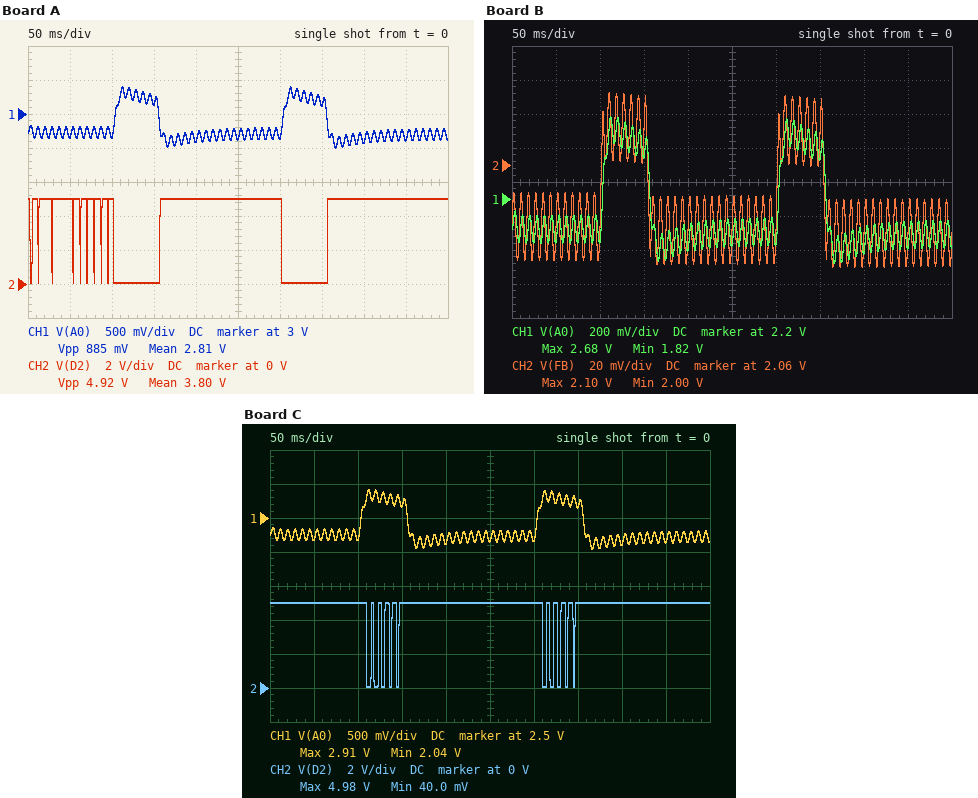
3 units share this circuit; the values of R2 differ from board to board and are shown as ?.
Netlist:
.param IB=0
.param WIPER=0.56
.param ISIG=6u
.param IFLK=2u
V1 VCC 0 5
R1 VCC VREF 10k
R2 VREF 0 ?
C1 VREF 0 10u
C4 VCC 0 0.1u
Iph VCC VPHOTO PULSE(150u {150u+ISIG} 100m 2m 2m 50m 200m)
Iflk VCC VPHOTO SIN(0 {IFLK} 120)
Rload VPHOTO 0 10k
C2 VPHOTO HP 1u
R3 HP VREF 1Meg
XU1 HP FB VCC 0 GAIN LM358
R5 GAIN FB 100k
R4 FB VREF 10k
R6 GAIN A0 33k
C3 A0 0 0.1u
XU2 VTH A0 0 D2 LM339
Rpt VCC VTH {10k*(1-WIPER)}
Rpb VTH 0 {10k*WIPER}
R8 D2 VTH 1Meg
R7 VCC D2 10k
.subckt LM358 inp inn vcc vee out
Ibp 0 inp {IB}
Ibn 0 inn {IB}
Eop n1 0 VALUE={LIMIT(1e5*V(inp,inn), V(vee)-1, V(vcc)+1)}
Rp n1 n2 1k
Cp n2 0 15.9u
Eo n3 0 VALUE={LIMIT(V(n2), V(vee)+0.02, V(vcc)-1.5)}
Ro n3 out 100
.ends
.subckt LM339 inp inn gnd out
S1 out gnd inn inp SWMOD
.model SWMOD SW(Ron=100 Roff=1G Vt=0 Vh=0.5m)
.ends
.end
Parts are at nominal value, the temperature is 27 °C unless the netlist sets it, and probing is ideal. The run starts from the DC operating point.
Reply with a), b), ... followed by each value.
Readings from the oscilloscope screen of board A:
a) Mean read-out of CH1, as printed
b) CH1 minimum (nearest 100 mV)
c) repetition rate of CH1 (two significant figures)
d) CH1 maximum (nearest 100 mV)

a) 2.81 V
b) 2.5 V
c) 5.0 Hz
d) 3.4 V
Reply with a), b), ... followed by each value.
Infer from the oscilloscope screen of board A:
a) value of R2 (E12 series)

a) 12 kΩ
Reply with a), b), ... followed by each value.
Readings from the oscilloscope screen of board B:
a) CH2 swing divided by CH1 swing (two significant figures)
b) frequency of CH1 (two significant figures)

a) 0.12
b) 5.0 Hz
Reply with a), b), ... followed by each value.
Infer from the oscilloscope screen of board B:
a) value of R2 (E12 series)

a) 6.8 kΩ
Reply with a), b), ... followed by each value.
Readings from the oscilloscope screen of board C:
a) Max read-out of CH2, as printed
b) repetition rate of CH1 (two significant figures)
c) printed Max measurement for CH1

a) 4.98 V
b) 5.0 Hz
c) 2.91 V
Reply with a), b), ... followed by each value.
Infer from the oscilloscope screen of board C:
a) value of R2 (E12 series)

a) 8.2 kΩ
